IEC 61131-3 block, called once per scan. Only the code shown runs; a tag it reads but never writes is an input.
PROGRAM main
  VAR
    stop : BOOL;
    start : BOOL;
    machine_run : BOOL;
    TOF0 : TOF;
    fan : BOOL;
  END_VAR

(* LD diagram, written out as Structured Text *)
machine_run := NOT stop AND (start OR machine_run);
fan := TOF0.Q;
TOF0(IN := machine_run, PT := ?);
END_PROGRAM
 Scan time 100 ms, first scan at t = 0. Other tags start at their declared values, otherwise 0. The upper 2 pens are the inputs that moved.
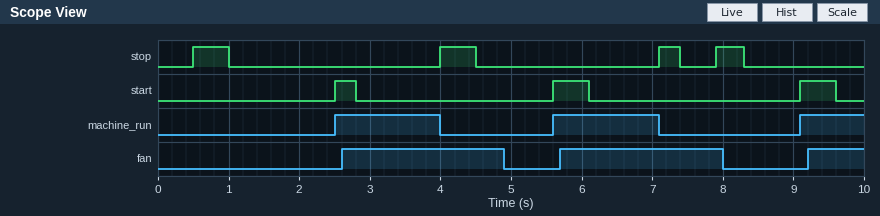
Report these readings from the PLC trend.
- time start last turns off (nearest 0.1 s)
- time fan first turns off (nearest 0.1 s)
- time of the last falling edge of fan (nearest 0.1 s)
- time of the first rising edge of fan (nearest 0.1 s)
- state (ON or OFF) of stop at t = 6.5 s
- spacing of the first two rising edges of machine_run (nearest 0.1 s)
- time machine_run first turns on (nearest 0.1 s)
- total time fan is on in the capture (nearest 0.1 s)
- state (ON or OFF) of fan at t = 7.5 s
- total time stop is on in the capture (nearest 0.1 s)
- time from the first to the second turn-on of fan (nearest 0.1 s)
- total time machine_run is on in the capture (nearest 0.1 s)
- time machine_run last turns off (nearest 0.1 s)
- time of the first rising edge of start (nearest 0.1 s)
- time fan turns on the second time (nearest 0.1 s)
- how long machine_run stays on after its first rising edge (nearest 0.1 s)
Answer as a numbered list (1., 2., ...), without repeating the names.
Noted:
1. 9.6 s
2. 4.9 s
3. 8.0 s
4. 2.6 s
5. OFF
6. 3.1 s
7. 2.5 s
8. 5.4 s
9. ON
10. 1.7 s
11. 3.1 s
12. 3.9 s
13. 7.1 s
14. 2.5 s
15. 5.7 s
16. 1.5 s
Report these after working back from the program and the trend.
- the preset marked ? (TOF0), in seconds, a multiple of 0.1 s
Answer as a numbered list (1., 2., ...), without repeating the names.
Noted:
1. 0.8 s
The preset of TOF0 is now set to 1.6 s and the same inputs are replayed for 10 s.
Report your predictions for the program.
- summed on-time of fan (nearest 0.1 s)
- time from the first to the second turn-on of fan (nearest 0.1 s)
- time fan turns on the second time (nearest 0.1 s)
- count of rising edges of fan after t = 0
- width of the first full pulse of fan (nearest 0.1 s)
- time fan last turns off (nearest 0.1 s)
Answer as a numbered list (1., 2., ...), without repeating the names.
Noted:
1. 7.0 s
2. 6.6 s
3. 9.2 s
4. 2
5. 6.2 s
6. 8.8 s
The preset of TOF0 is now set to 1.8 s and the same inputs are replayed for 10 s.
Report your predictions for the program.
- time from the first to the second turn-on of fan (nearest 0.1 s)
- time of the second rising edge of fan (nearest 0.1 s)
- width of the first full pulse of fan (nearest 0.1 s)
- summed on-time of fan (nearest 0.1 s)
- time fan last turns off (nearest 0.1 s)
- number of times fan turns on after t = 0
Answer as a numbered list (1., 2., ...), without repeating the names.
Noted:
1. 6.6 s
2. 9.2 s
3. 6.4 s
4. 7.2 s
5. 9.0 s
6. 2
